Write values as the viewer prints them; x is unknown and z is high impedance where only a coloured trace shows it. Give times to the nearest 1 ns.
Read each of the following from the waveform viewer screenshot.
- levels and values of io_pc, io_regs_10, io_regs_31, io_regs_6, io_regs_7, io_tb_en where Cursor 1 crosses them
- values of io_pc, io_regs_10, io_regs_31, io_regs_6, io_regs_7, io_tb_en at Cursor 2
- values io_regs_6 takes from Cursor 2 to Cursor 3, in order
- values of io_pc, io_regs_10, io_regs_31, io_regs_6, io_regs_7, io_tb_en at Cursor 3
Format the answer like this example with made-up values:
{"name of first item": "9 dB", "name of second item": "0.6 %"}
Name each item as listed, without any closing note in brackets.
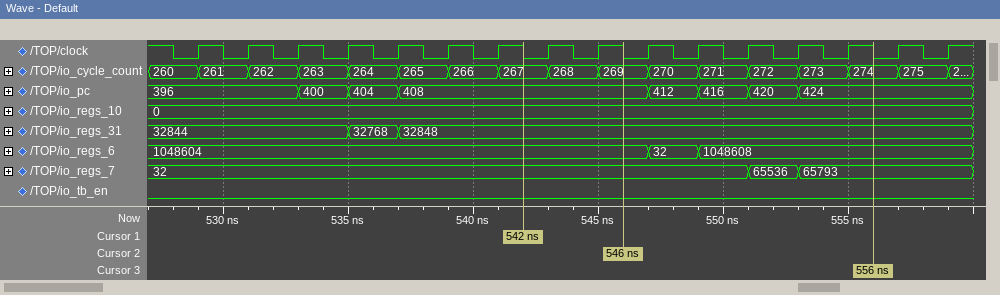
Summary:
{"levels and values of io_pc, io_regs_10, io_regs_31, io_regs_6, io_regs_7, io_tb_en where Cursor 1 crosses them": "io_pc=408, io_regs_10=0, io_regs_31=32848, io_regs_6=1048604, io_regs_7=32, io_tb_en=0", "values of io_pc, io_regs_10, io_regs_31, io_regs_6, io_regs_7, io_tb_en at Cursor 2": "io_pc=408, io_regs_10=0, io_regs_31=32848, io_regs_6=1048604, io_regs_7=32, io_tb_en=0", "values io_regs_6 takes from Cursor 2 to Cursor 3, in order": "1048604, 32, 1048608", "values of io_pc, io_regs_10, io_regs_31, io_regs_6, io_regs_7, io_tb_en at Cursor 3": "io_pc=424, io_regs_10=0, io_regs_31=32848, io_regs_6=1048608, io_regs_7=65793, io_tb_en=0"}
